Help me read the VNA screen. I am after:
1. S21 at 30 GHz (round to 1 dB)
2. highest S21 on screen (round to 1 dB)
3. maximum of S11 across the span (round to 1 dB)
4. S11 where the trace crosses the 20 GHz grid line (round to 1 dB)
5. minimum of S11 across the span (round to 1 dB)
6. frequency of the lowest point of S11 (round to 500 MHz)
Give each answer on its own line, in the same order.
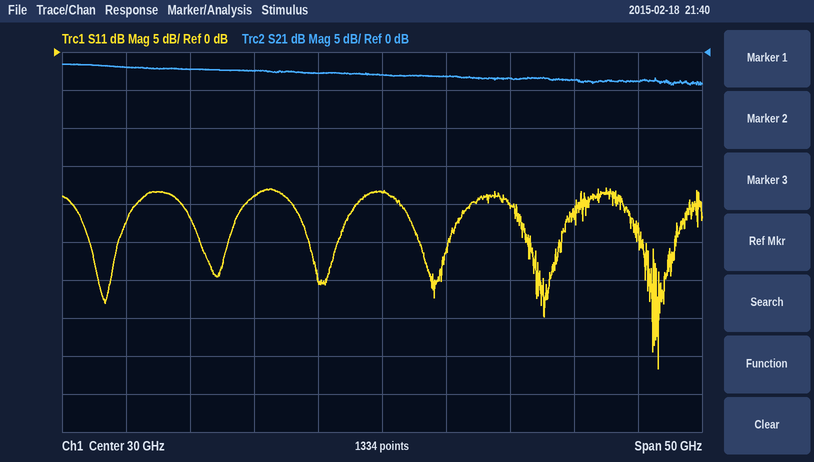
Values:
-3 dB
-2 dB
-18 dB
-19 dB
-42 dB
51.5 GHz
